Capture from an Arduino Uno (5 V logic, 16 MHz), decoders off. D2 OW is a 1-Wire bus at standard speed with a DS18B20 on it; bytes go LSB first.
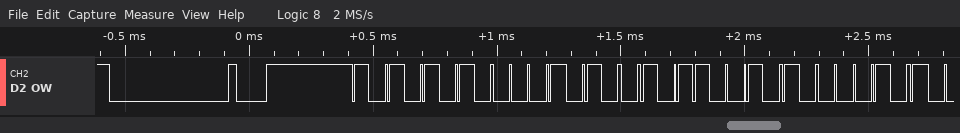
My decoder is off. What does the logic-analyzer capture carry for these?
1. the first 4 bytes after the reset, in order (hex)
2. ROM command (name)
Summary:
55 28 4D A1
Match ROM
